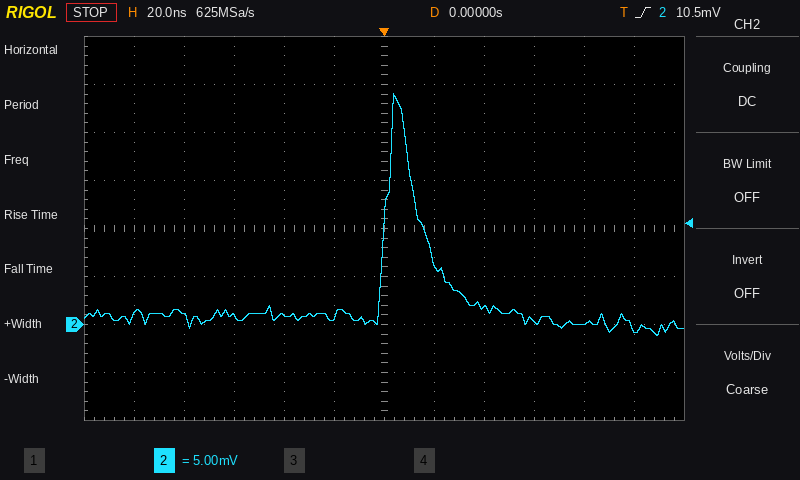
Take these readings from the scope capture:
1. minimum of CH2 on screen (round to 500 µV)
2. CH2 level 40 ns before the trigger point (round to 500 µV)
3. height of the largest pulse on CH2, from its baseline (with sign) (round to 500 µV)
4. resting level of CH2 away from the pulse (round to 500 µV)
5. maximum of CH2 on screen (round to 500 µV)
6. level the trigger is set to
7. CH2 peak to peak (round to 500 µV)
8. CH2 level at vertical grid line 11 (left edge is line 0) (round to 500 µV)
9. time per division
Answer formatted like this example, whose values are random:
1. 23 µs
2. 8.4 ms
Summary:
1. -1.0 mV
2. 1.0 mV
3. +23.0 mV
4. 1.0 mV
5. 24.0 mV
6. 10.5 mV
7. 25.0 mV
8. -500 µV
9. 20 ns
